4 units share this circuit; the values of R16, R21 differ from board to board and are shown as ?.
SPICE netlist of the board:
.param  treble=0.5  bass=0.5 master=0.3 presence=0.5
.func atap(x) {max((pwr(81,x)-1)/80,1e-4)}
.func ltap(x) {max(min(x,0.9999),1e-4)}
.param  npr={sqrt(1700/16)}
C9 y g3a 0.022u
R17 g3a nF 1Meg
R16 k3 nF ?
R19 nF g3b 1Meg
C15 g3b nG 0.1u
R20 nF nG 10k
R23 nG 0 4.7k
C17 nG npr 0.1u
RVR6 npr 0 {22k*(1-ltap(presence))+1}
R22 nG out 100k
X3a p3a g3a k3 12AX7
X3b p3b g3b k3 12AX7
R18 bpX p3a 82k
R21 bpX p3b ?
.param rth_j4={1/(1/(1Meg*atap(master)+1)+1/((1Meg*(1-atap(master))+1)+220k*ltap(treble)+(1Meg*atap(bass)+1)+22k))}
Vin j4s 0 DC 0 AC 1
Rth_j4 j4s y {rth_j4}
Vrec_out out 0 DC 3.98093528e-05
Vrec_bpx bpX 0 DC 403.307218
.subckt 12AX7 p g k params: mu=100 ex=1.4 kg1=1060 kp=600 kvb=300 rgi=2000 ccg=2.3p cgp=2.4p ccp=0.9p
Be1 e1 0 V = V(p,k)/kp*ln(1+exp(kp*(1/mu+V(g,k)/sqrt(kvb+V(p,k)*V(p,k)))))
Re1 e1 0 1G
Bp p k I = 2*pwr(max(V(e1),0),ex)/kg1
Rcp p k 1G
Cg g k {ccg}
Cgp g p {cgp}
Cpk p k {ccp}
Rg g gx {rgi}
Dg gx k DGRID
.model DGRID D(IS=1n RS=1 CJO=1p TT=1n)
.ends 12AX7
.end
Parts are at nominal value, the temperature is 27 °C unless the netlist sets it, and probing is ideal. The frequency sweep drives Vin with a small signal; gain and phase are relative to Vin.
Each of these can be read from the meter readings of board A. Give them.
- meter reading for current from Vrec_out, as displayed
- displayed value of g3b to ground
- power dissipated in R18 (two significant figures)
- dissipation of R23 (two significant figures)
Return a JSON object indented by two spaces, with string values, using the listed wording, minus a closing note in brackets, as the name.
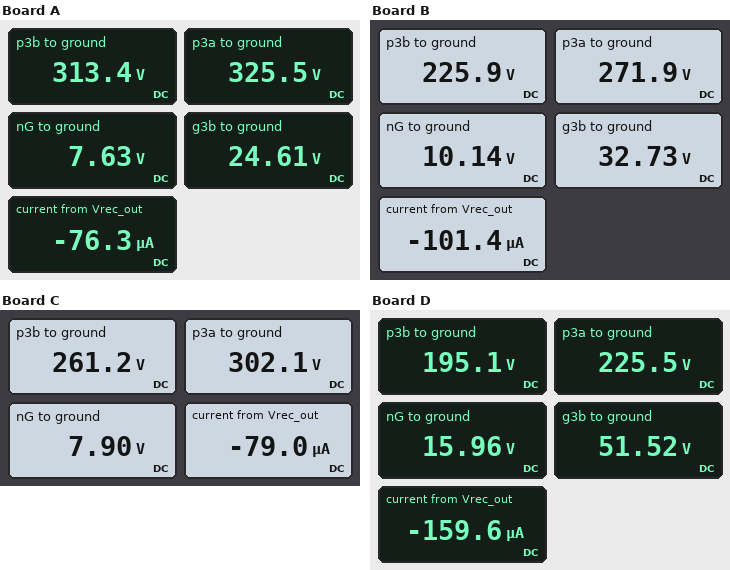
{
  "meter reading for current from Vrec_out, as displayed": "-76.3 µA",
  "displayed value of g3b to ground": "24.61 V",
  "power dissipated in R18": "74 mW",
  "dissipation of R23": "12 mW"
}
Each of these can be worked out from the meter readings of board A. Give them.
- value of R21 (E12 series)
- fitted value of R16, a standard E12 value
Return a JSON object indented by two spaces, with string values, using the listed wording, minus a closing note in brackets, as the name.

{
  "value of R21": "120 kΩ",
  "fitted value of R16, a standard E12 value": "1.5 kΩ"
}
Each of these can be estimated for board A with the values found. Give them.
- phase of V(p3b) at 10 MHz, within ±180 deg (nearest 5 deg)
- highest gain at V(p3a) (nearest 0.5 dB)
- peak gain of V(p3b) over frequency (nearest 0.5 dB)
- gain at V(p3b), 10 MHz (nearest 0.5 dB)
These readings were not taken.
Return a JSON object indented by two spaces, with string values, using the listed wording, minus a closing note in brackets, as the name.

{
  "phase of V(p3b) at 10 MHz, within ±180 deg": "-70 deg",
  "highest gain at V(p3a)": "26.5 dB",
  "peak gain of V(p3b) over frequency": "28.0 dB",
  "gain at V(p3b), 10 MHz": "-16.5 dB"
}
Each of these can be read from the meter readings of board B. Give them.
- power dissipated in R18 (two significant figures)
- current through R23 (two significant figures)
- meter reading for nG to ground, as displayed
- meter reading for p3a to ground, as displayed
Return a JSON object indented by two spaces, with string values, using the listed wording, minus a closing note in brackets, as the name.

{
  "power dissipated in R18": "210 mW",
  "current through R23": "2.2 mA",
  "meter reading for nG to ground, as displayed": "10.14 V",
  "meter reading for p3a to ground, as displayed": "271.9 V"
}
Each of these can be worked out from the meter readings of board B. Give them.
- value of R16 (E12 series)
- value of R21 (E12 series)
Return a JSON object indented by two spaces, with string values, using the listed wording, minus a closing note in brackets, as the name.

{
  "value of R16": "680 Ω",
  "value of R21": "270 kΩ"
}
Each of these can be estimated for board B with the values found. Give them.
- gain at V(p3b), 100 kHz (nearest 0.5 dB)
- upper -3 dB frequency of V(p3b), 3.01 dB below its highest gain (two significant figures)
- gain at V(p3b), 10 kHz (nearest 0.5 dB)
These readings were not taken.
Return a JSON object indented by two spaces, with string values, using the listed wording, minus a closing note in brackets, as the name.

{
  "gain at V(p3b), 100 kHz": "28.5 dB",
  "upper -3 dB frequency of V(p3b), 3.01 dB below its highest gain": "89 kHz",
  "gain at V(p3b), 10 kHz": "32.0 dB"
}
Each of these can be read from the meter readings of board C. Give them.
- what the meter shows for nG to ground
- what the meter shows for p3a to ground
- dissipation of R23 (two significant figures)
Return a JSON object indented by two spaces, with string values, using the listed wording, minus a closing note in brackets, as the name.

{
  "what the meter shows for nG to ground": "7.90 V",
  "what the meter shows for p3a to ground": "302.1 V",
  "dissipation of R23": "13 mW"
}
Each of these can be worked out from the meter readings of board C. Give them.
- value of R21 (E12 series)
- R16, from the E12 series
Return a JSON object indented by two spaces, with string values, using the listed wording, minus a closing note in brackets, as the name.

{
  "value of R21": "270 kΩ",
  "R16, from the E12 series": "1.2 kΩ"
}
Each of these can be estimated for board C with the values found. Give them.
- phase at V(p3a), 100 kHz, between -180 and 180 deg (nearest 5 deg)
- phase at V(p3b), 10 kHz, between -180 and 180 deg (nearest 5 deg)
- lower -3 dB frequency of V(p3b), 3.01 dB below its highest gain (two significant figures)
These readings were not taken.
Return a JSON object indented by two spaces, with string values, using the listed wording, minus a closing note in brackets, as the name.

{
  "phase at V(p3a), 100 kHz, between -180 and 180 deg": "135 deg",
  "phase at V(p3b), 10 kHz, between -180 and 180 deg": "-5 deg",
  "lower -3 dB frequency of V(p3b), 3.01 dB below its highest gain": "3.6 Hz"
}
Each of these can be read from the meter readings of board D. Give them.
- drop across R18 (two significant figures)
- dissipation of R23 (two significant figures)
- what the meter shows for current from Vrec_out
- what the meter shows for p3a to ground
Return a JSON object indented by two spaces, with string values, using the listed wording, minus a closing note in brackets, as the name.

{
  "drop across R18": "180 V",
  "dissipation of R23": "54 mW",
  "what the meter shows for current from Vrec_out": "-159.6 µA",
  "what the meter shows for p3a to ground": "225.5 V"
}
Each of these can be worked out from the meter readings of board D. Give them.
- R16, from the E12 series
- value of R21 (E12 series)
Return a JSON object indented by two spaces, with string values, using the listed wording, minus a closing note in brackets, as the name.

{
  "R16, from the E12 series": "180 Ω",
  "value of R21": "150 kΩ"
}
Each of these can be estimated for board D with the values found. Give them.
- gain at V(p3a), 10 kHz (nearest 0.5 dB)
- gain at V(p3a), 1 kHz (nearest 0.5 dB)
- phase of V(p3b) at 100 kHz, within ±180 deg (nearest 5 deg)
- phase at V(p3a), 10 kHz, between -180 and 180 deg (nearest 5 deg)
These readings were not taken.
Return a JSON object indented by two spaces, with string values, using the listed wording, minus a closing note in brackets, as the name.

{
  "gain at V(p3a), 10 kHz": "27.5 dB",
  "gain at V(p3a), 1 kHz": "27.5 dB",
  "phase of V(p3b) at 100 kHz, within ±180 deg": "-60 deg",
  "phase at V(p3a), 10 kHz, between -180 and 180 deg": "170 deg"
}
